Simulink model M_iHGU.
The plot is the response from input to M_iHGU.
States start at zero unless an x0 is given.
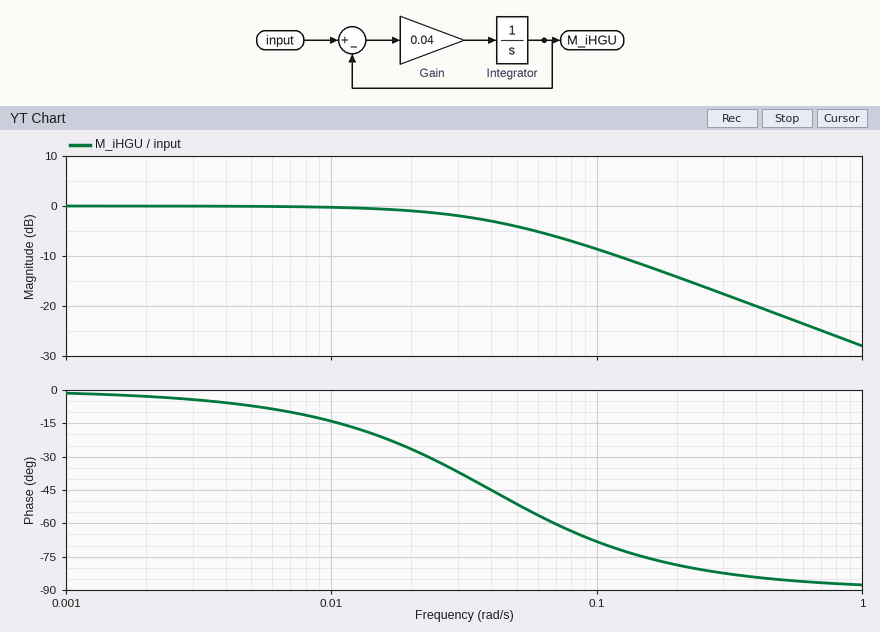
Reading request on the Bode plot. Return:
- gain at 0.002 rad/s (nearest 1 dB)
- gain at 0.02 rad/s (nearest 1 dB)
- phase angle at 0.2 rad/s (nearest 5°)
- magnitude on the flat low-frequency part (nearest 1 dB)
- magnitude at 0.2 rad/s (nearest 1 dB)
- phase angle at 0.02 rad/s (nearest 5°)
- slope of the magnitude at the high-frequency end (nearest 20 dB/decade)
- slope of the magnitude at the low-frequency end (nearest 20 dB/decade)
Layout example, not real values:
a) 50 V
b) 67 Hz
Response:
a) 0 dB
b) -1 dB
c) -80°
d) 0 dB
e) -14 dB
f) -25°
g) -20 dB/decade
h) 0 dB/decade
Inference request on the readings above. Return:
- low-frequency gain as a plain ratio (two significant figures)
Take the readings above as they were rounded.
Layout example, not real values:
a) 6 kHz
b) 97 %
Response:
a) 1.0
